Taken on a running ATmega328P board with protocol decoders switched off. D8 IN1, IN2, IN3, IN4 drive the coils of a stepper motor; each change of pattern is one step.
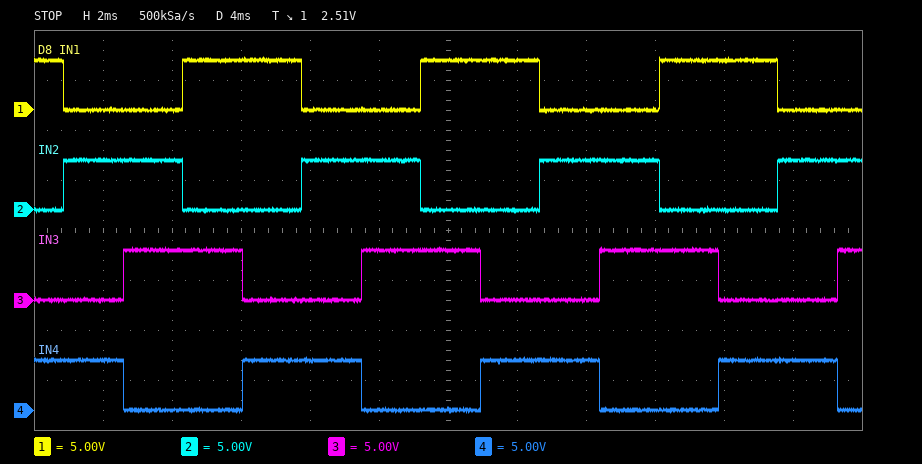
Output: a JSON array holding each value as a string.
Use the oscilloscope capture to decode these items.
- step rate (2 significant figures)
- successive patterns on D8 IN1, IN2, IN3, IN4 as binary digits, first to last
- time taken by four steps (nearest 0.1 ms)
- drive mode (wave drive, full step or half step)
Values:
["580 steps/s", "1001 0101 0110 1010 1001 0101 0110 1010 1001 0101 0110 1010 1001 0101 0110", "6.9 ms", "full step"]
